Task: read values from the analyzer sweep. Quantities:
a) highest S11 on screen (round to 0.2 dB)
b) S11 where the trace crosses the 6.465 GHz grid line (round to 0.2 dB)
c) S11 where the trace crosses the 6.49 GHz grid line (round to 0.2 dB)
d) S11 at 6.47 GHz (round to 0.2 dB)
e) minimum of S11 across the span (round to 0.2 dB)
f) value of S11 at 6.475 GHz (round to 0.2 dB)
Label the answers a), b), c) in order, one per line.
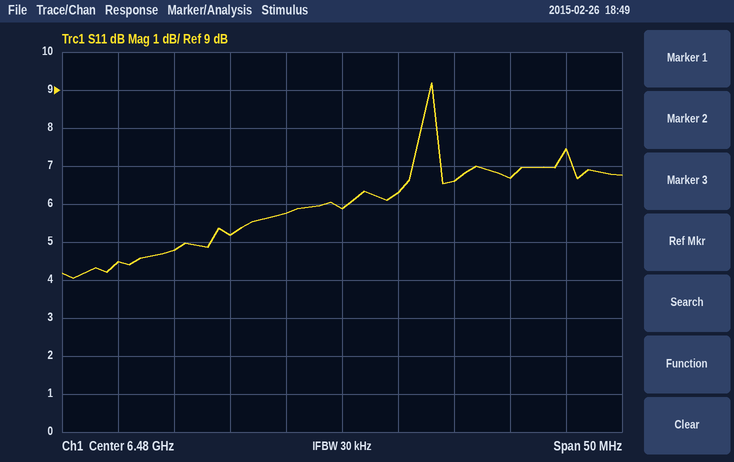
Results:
a) 9.2 dB
b) 4.8 dB
c) 6.6 dB
d) 5.2 dB
e) 4.0 dB
f) 5.8 dB
